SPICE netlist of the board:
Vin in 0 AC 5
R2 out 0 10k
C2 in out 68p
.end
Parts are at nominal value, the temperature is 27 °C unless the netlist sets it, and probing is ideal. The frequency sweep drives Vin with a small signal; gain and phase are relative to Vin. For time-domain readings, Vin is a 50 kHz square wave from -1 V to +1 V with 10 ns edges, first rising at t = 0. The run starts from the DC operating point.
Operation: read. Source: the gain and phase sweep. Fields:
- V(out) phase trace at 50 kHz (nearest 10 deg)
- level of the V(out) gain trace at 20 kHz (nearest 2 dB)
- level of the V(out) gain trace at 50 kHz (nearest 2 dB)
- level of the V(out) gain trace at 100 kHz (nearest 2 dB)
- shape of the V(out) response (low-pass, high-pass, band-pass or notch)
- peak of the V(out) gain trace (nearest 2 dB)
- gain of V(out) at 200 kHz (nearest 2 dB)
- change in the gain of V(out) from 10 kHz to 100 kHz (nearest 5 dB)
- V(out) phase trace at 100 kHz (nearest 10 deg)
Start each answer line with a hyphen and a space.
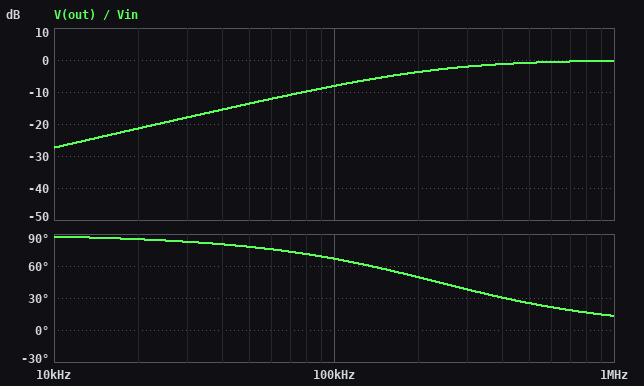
- 80 deg
- -22 dB
- -14 dB
- -8 dB
- high-pass
- 0 dB
- -4 dB
- 20 dB
- 70 deg
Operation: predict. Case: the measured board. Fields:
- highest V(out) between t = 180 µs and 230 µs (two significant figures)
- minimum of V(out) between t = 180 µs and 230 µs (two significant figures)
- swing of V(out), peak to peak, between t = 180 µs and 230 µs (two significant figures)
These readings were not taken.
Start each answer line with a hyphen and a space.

- 2.0 V
- -2.0 V
- 4.0 V
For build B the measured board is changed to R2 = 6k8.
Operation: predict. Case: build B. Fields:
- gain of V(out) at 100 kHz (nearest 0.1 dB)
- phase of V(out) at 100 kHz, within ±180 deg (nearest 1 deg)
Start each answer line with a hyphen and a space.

- -11.1 dB
- 74 deg
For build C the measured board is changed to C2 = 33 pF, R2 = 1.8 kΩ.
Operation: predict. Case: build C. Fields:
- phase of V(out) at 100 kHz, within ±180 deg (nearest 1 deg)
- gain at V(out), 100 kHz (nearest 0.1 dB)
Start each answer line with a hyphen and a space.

- 88 deg
- -28.6 dB
